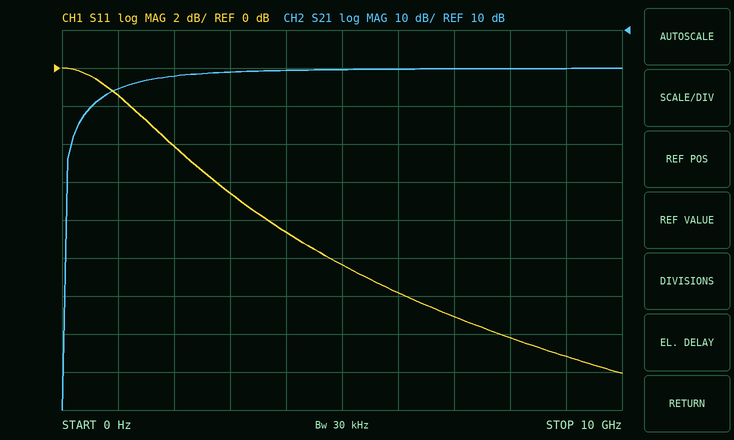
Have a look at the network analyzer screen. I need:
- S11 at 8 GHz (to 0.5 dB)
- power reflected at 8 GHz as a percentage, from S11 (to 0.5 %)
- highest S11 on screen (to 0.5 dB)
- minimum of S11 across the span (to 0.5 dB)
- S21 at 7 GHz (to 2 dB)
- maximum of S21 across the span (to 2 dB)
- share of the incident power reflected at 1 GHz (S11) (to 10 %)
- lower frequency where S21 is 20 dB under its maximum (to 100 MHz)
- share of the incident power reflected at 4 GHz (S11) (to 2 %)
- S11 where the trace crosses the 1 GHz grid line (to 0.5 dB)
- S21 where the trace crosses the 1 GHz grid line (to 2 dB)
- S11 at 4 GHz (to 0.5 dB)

-14.0 dB
4.0 %
0.0 dB
-16.0 dB
0 dB
0 dB
70 %
200 MHz
14 %
-1.5 dB
-6 dB
-8.5 dB
